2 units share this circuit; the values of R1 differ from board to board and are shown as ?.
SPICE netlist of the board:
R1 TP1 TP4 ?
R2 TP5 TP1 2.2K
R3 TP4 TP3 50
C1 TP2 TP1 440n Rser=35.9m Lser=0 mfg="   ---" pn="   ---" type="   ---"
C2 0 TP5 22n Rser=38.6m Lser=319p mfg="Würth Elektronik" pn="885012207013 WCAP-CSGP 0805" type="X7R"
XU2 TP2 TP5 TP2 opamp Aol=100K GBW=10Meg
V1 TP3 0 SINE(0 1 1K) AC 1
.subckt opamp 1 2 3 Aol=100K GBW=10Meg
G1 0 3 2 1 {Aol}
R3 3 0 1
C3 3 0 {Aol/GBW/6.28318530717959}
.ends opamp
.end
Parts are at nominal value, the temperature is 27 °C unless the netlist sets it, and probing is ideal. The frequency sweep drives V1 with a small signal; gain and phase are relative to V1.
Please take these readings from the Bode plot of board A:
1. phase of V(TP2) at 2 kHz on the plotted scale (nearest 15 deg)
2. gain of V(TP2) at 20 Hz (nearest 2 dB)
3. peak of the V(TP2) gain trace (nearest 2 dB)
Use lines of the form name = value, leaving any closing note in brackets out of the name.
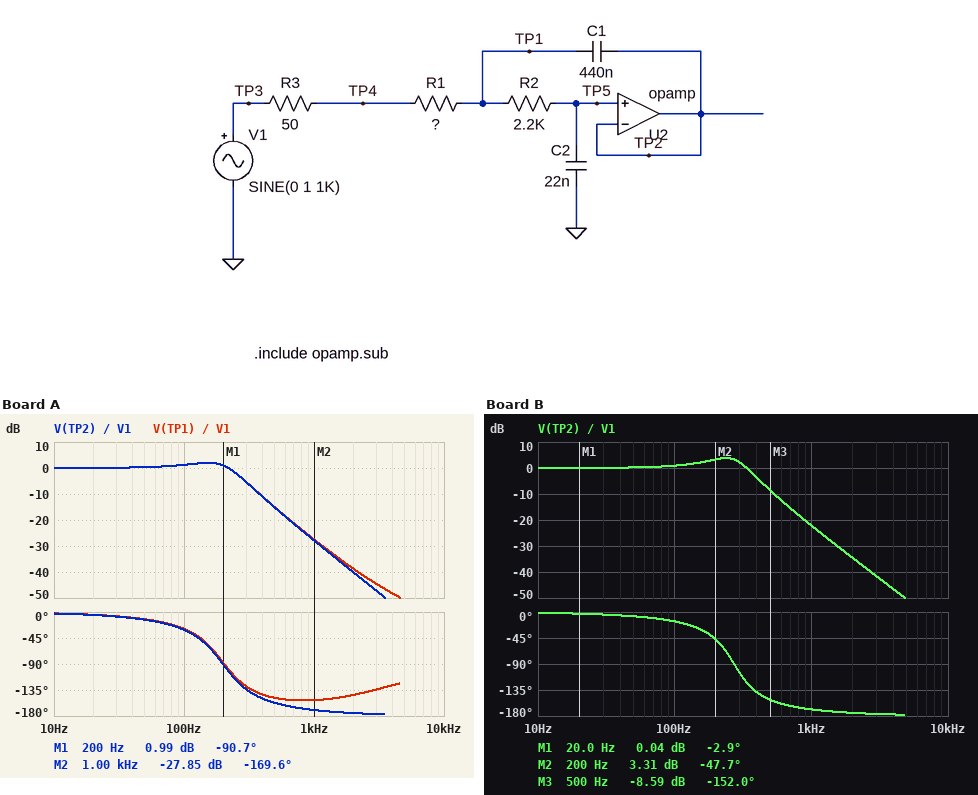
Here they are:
phase of V(TP2) at 2 kHz on the plotted scale = -180 deg
gain of V(TP2) at 20 Hz = 0 dB
peak of the V(TP2) gain trace = 2 dB
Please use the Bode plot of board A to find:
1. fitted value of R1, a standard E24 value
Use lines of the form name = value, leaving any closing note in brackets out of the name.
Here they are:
fitted value of R1, a standard E24 value = 30 kΩ
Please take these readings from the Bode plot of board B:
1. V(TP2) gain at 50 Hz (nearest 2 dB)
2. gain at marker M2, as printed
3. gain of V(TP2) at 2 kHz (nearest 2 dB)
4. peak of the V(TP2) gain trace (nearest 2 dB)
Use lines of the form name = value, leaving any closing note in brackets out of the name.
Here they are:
V(TP2) gain at 50 Hz = 0 dB
gain at marker M2, as printed = 3.31 dB
gain of V(TP2) at 2 kHz = -34 dB
peak of the V(TP2) gain trace = 4 dB
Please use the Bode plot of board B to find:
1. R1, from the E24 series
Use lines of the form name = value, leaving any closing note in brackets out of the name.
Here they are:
R1, from the E24 series = 16 kΩ
